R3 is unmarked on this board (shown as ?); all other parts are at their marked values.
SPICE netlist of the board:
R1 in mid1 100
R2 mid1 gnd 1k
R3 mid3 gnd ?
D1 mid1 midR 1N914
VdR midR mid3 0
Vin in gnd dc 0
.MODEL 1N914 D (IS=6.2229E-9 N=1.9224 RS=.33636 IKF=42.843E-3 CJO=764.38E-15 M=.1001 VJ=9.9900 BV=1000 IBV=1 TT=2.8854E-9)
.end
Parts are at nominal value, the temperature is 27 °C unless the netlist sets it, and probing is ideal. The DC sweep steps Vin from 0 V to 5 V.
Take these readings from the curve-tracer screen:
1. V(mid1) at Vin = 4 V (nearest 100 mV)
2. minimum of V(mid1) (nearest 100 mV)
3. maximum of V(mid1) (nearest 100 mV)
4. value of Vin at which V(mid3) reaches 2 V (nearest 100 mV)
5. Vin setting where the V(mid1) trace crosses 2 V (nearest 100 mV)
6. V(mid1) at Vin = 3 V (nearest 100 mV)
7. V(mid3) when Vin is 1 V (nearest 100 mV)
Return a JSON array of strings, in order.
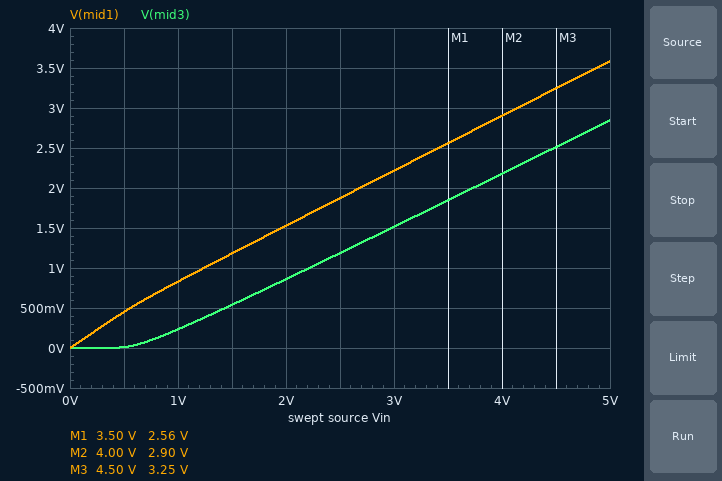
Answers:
["2.9 V", "0 V", "3.6 V", "3.7 V", "2.7 V", "2.2 V", "200 mV"]
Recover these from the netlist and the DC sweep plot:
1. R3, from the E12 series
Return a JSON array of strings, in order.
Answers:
["270 Ω"]
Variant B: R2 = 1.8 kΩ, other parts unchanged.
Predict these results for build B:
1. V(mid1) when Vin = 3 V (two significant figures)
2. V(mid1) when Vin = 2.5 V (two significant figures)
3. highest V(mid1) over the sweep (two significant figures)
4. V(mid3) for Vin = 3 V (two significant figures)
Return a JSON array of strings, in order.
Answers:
["2.3 V", "1.9 V", "3.7 V", "1.6 V"]
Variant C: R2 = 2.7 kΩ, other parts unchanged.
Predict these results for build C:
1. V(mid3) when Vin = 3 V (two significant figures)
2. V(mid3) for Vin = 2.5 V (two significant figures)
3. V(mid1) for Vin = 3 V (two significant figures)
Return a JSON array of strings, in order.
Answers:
["1.6 V", "1.3 V", "2.3 V"]
